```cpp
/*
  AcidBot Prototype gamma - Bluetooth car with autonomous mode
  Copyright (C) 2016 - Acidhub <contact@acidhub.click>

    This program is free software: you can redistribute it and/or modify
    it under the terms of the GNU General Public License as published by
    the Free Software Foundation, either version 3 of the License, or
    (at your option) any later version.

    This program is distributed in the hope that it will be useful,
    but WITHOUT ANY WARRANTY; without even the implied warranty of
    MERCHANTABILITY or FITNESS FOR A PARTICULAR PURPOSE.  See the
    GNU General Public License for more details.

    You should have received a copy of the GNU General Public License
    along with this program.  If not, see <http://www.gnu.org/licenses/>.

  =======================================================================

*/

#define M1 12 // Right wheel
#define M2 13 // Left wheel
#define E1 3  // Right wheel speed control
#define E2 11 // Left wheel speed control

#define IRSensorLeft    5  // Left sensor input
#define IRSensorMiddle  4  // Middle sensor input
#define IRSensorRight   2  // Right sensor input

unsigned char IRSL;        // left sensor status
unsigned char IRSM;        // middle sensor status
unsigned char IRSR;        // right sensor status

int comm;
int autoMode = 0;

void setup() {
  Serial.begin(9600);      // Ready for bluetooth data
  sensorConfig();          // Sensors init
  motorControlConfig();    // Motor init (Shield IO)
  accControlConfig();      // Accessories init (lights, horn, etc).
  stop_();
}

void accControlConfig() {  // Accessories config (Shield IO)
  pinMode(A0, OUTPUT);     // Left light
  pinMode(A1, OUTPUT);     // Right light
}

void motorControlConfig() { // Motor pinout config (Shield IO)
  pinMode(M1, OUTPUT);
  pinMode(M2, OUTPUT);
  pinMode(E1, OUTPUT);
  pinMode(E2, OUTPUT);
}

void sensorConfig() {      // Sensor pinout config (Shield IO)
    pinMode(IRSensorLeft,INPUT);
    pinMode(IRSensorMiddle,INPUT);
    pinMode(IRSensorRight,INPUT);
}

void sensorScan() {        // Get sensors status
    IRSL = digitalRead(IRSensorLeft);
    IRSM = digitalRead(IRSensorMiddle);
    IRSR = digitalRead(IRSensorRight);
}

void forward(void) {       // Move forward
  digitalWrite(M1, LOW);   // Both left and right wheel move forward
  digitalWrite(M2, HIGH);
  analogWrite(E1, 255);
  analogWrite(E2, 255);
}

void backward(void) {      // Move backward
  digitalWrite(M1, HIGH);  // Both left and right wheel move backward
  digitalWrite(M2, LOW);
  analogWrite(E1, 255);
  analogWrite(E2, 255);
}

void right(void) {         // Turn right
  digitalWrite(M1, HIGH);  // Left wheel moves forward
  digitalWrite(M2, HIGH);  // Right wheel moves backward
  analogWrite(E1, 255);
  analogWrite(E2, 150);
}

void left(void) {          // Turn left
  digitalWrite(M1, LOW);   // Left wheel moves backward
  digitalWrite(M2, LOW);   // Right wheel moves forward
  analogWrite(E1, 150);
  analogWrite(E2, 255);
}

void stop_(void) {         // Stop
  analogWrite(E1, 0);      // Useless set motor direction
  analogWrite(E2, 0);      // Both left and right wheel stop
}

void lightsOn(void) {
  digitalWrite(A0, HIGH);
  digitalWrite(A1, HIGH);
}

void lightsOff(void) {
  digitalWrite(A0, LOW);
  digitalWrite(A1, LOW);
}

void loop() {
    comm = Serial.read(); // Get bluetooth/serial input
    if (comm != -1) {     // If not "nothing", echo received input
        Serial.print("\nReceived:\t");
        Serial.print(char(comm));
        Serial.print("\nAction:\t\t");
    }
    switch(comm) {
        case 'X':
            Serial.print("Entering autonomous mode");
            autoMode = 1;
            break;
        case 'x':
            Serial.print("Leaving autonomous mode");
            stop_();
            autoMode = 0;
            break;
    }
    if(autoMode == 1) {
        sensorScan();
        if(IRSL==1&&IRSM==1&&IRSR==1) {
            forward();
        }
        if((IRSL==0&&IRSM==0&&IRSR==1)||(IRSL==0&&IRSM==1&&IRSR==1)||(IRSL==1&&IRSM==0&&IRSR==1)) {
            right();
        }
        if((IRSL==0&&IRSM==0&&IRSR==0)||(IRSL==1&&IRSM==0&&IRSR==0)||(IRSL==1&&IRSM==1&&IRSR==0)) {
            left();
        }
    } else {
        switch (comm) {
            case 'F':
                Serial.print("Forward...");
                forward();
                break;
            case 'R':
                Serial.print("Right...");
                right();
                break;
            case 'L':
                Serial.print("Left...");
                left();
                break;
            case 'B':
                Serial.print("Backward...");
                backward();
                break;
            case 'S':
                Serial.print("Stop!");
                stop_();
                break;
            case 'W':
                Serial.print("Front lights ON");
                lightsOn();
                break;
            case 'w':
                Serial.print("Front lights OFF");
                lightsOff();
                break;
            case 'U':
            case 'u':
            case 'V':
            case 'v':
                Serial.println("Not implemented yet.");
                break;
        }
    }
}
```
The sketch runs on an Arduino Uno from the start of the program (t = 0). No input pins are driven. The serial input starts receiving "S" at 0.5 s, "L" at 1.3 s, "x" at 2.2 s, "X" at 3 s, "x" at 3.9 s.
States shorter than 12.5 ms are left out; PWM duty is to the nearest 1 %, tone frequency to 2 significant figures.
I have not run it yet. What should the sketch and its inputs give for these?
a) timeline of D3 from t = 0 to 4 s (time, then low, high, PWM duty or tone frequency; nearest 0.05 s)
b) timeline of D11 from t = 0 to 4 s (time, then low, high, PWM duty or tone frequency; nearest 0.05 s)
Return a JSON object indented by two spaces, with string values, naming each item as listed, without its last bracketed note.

{
  "timeline of D3 from t = 0 to 4 s": "0 s low; 1.3 s PWM 59 %; 2.2 s low; 3 s PWM 59 %; 3.9 s low",
  "timeline of D11 from t = 0 to 4 s": "0 s low; 1.3 s high; 2.2 s low; 3 s high; 3.9 s low"
}
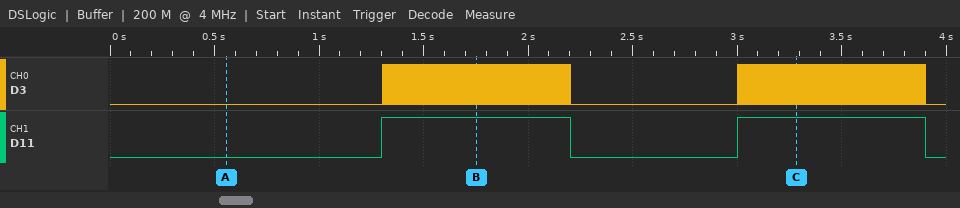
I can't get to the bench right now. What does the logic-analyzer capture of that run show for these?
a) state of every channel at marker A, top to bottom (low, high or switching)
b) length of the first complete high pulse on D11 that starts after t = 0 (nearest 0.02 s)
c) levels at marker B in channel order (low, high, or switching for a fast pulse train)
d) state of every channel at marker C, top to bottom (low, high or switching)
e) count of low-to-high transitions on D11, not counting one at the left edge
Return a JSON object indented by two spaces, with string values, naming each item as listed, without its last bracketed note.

{
  "state of every channel at marker A, top to bottom": "D3 low, D11 low",
  "length of the first complete high pulse on D11 that starts after t = 0": "0.90 s",
  "levels at marker B in channel order": "D3 switching, D11 high",
  "state of every channel at marker C, top to bottom": "D3 switching, D11 high",
  "count of low-to-high transitions on D11, not counting one at the left edge": "2"
}
